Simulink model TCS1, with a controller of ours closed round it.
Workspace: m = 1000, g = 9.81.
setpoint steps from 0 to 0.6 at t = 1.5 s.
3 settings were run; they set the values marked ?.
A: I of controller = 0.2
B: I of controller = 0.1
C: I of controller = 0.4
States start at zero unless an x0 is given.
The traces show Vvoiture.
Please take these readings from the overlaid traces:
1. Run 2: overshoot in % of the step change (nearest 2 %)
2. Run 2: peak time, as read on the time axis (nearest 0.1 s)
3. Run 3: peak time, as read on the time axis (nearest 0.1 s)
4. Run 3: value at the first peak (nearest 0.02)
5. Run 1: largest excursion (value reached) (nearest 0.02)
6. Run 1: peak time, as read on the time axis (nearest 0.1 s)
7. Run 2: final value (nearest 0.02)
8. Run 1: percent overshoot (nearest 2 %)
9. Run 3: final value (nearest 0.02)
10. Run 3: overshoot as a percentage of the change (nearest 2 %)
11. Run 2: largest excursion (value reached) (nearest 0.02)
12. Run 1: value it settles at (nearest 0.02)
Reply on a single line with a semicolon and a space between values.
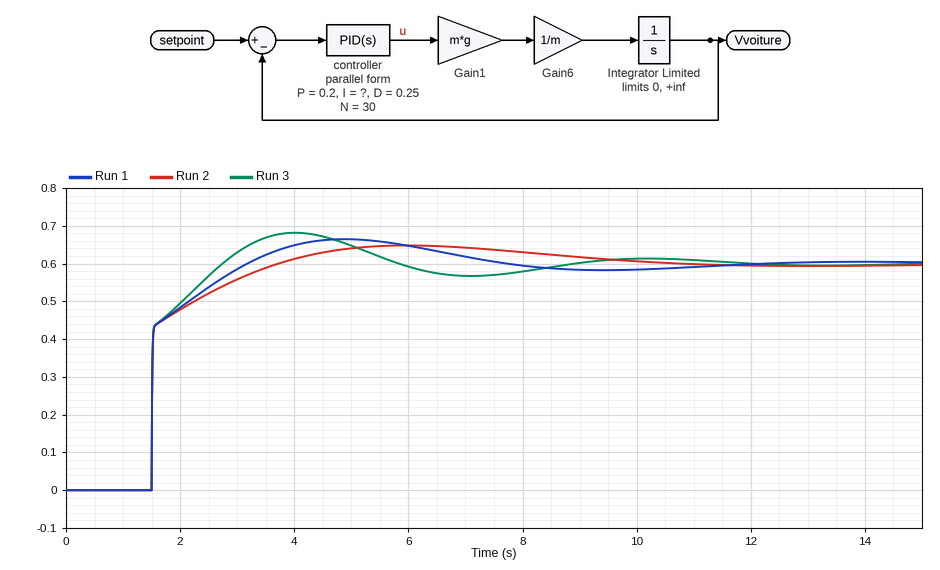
8 %; 6.0 s; 4.0 s; 0.68; 0.66; 4.9 s; 0.60; 10 %; 0.60; 14 %; 0.64; 0.60
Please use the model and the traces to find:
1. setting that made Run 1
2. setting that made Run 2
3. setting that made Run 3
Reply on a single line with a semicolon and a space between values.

A; B; C
